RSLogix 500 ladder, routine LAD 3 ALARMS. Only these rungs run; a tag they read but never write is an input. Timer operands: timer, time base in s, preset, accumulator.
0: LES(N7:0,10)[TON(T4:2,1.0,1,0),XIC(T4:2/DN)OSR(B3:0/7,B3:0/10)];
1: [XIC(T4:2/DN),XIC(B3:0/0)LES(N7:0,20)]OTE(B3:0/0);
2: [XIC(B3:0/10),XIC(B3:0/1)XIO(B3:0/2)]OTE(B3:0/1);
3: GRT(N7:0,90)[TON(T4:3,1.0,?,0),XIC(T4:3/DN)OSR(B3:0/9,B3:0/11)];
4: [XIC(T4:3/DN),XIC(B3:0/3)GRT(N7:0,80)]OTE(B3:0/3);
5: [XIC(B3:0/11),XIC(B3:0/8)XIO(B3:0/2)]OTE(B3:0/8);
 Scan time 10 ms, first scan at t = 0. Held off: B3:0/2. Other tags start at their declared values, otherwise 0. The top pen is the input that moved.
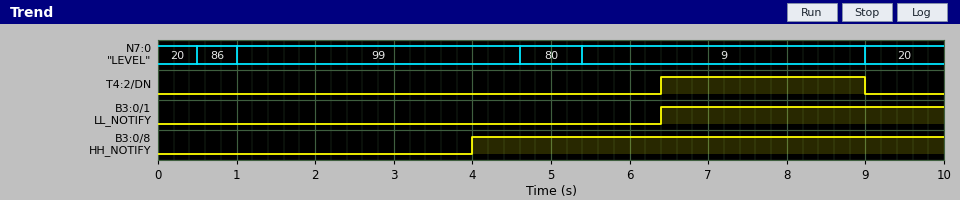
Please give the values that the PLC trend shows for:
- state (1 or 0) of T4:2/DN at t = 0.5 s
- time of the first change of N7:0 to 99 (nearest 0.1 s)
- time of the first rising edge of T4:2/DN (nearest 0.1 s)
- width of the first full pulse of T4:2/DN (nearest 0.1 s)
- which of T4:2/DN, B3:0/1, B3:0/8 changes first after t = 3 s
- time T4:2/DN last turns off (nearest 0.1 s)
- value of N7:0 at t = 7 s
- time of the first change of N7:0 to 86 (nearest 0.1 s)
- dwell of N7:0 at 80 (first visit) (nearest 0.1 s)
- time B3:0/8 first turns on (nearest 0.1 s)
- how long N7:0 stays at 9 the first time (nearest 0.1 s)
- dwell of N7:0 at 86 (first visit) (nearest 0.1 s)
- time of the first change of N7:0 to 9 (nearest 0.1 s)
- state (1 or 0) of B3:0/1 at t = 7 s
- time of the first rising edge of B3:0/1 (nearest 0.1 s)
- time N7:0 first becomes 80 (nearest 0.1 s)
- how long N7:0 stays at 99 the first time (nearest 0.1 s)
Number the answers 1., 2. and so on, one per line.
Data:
1. 0
2. 1.0 s
3. 6.4 s
4. 2.6 s
5. B3:0/8
6. 9.0 s
7. 9
8. 0.5 s
9. 0.8 s
10. 4.0 s
11. 3.6 s
12. 0.5 s
13. 5.4 s
14. 1
15. 6.4 s
16. 4.6 s
17. 3.6 s
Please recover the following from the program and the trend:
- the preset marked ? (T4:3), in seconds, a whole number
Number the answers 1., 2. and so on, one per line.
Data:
1. 3 s
